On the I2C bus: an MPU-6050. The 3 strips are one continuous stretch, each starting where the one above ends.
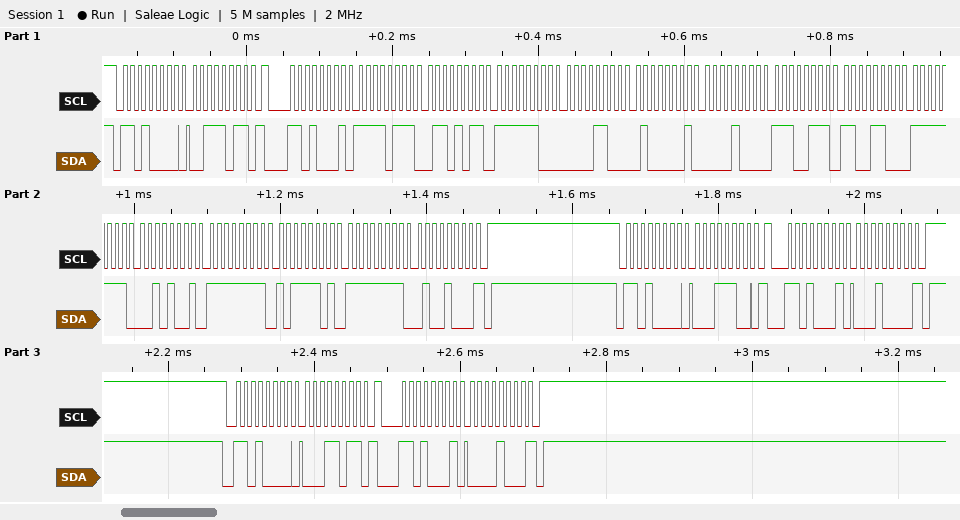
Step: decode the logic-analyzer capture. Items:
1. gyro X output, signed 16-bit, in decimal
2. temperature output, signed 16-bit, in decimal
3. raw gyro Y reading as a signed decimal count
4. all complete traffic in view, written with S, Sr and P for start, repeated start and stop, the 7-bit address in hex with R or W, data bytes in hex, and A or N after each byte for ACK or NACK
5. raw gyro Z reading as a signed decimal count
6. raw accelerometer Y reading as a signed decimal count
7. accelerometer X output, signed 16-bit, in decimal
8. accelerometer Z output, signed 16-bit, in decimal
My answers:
-215
-6196
-67
S 68W A 3B A Sr 68R A F7 A 6B A FC A 0C A 41 A 08 A E7 A CC A FF A 29 A FF A BD A FF A 48 N P S 68W A 1C A Sr 68R A 10 N P S 68W A 1B A Sr 68R A 08 N P
-184
-1012
-2197
16648
